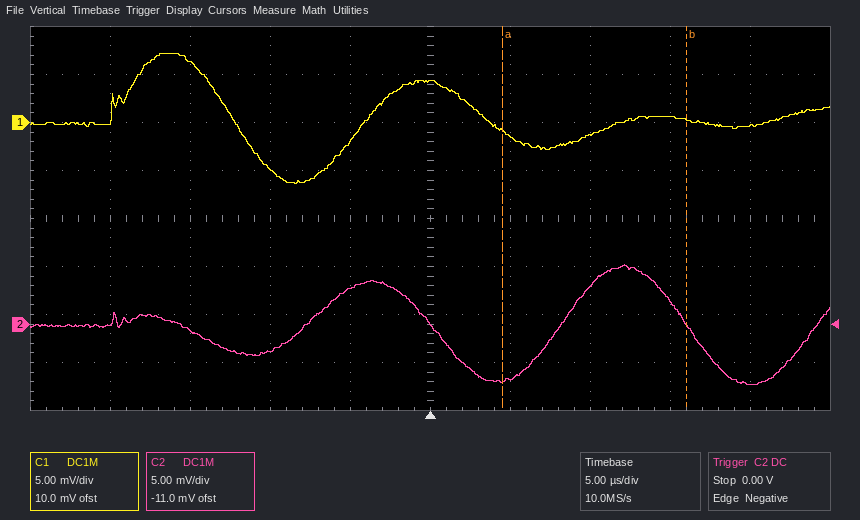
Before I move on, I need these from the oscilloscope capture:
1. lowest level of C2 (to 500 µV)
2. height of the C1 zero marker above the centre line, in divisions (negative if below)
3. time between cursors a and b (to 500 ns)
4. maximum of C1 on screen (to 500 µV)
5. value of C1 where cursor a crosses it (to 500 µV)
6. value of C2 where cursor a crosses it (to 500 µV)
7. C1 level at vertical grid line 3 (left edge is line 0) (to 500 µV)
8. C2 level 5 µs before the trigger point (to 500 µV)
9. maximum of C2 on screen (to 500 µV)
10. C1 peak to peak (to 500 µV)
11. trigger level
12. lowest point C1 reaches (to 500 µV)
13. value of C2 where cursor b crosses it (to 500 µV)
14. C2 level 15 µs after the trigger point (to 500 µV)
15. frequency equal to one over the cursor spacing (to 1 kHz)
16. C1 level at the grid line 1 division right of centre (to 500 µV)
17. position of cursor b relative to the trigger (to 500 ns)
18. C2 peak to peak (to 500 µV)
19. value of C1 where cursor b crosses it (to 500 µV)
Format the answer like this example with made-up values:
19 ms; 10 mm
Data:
-6.5 mV; +2.0 div; 11.5 µs; 7.0 mV; -1.0 mV; -6.0 mV; -5.0 mV; 3.5 mV; 6.0 mV; 13.5 mV; 0.00 V; -6.5 mV; 0.0 mV; 2.5 mV; 87 kHz; -1.5 mV; +16.0 µs; 12.5 mV; 500 µV
